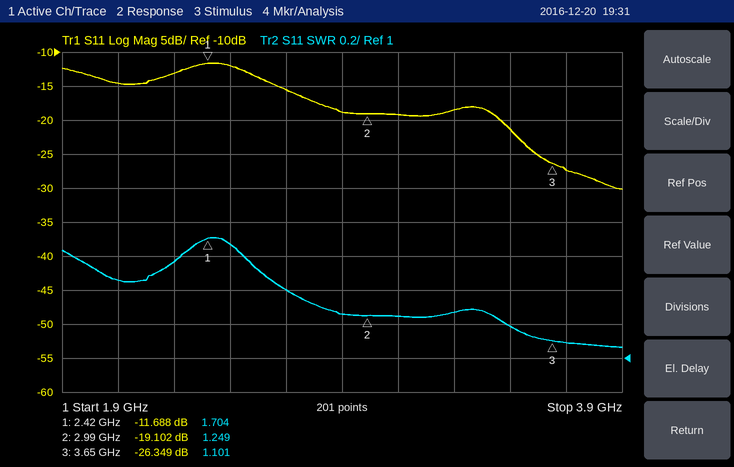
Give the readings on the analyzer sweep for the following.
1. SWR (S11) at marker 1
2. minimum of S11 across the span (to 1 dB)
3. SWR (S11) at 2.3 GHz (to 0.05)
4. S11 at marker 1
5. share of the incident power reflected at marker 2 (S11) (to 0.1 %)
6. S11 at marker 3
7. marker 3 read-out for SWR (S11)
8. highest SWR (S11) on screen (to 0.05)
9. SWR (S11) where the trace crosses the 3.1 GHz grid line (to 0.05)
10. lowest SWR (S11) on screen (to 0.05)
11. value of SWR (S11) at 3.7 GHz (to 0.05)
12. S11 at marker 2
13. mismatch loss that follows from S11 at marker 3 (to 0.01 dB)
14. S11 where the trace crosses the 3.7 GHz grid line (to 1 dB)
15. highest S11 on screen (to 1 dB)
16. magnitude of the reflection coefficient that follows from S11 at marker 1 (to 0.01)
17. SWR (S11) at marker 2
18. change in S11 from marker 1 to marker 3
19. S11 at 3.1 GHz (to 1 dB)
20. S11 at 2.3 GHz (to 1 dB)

1.704
-30 dB
1.55
-11.688 dB
1.2 %
-26.349 dB
1.101
1.70
1.25
1.05
1.10
-19.102 dB
0.01 dB
-27 dB
-12 dB
0.26
1.249
-14.661 dB
-19 dB
-13 dB
